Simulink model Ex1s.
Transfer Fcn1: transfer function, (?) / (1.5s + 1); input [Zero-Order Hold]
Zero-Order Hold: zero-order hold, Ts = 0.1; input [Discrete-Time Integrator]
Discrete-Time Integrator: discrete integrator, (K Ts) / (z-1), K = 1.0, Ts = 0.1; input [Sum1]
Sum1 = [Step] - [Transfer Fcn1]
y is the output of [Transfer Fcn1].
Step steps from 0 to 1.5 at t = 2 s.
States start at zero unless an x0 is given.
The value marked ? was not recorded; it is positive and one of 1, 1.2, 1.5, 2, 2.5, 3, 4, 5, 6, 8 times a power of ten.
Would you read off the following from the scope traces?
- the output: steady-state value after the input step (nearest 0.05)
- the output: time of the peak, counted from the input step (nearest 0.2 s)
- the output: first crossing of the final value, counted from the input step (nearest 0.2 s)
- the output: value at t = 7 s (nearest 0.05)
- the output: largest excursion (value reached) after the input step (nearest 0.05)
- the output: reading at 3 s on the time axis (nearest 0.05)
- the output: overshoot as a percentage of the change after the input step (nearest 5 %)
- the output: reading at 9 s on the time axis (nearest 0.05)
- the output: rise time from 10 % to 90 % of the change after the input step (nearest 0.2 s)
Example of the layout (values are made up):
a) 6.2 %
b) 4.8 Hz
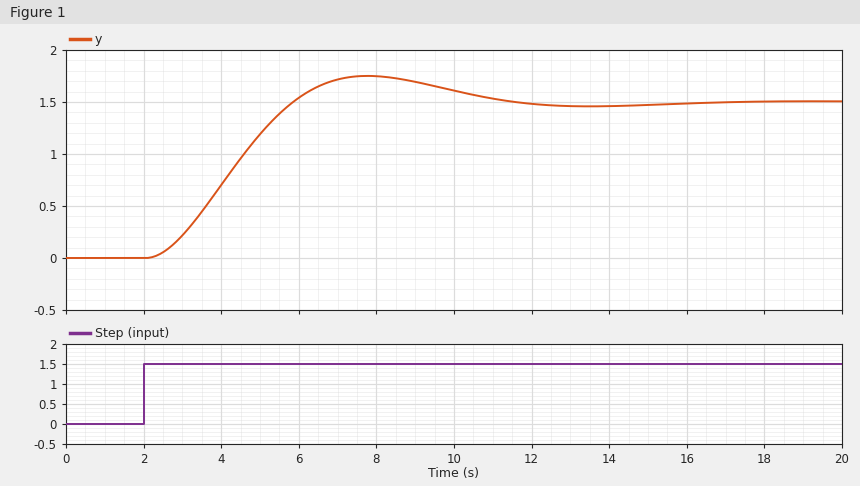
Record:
a) 1.50
b) 5.8 s
c) 3.8 s
d) 1.70
e) 1.75
f) 0.20
g) 15 %
h) 1.70
i) 2.6 s
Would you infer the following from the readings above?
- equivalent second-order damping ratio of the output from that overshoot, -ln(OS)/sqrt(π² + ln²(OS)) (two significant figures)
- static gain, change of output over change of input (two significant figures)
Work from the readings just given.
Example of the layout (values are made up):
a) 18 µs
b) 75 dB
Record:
a) 0.52
b) 1.0
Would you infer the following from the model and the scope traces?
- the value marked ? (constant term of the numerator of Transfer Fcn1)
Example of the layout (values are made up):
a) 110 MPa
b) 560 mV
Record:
a) 0.6
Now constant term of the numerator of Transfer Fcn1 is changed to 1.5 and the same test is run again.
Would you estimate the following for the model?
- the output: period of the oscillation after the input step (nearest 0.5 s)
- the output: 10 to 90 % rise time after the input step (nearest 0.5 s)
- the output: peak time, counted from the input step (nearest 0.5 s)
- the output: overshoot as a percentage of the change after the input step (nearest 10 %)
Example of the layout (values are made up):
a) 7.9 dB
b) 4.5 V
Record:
a) 6.5 s
b) 1.5 s
c) 3.5 s
d) 40 %
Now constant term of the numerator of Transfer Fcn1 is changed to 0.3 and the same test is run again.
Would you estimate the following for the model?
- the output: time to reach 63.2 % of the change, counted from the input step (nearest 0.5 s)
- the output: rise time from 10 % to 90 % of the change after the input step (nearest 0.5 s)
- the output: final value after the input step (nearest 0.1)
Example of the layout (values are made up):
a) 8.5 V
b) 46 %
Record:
a) 4.0 s
b) 5.0 s
c) 1.5
